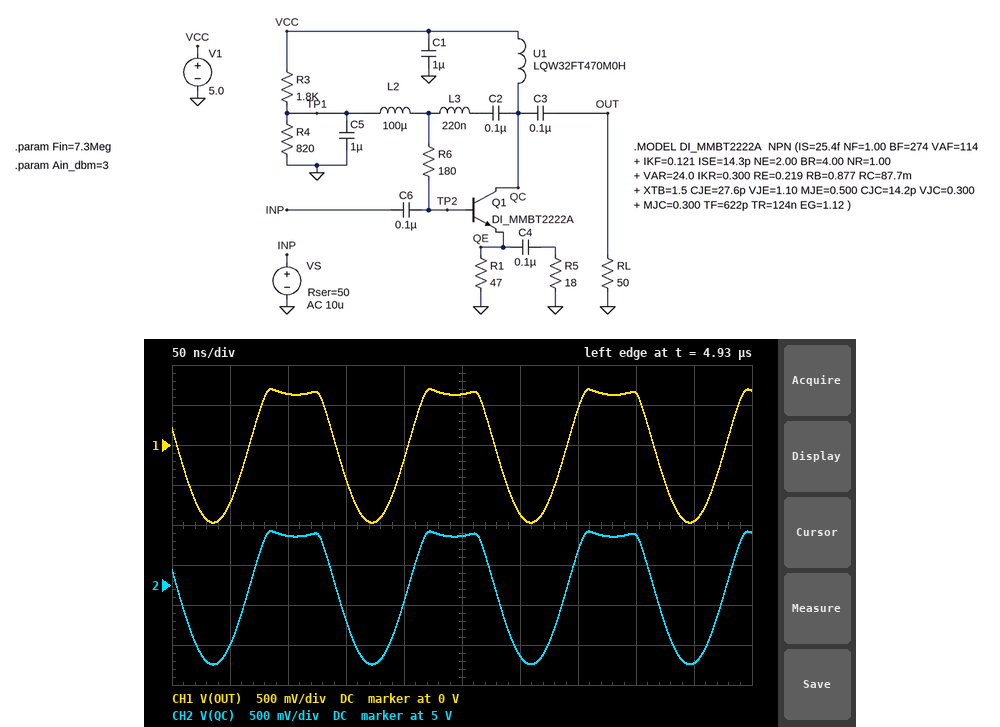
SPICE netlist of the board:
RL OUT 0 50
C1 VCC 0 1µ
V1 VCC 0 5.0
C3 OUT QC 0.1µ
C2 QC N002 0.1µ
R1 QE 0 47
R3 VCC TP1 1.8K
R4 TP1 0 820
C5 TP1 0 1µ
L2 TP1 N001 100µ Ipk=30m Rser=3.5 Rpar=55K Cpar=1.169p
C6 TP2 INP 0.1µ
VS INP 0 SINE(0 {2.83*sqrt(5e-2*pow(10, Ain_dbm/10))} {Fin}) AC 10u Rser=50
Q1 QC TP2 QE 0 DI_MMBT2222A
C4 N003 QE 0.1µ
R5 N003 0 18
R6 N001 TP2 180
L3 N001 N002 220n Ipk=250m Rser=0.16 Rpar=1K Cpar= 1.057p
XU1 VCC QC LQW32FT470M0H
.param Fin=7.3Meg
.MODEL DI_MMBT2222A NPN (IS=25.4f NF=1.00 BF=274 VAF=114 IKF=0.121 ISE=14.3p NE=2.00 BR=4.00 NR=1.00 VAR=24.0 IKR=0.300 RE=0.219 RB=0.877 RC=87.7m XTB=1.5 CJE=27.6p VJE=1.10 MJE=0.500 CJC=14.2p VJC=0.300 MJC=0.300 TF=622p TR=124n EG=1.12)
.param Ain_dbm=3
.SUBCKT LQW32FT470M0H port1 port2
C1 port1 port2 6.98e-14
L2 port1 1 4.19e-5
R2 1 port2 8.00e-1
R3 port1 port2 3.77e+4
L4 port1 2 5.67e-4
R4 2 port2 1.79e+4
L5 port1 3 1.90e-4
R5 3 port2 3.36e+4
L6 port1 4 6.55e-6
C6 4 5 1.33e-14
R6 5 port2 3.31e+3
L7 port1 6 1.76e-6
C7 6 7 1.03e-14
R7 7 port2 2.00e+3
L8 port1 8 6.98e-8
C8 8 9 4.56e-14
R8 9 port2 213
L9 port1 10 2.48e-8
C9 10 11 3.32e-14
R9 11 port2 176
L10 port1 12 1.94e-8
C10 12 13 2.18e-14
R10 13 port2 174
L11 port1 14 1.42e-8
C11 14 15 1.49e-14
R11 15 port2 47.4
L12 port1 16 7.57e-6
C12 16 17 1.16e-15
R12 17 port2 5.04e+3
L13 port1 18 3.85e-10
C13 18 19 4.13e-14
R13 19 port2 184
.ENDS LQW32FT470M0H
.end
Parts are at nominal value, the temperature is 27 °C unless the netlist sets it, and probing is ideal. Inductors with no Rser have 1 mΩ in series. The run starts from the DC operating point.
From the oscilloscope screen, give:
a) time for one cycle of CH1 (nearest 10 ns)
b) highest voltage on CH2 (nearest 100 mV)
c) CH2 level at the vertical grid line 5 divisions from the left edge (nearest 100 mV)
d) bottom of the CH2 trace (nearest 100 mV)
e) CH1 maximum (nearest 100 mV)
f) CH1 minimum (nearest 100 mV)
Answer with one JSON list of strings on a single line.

["140 ns", "5.7 V", "5.6 V", "4.0 V", "700 mV", "-1.0 V"]
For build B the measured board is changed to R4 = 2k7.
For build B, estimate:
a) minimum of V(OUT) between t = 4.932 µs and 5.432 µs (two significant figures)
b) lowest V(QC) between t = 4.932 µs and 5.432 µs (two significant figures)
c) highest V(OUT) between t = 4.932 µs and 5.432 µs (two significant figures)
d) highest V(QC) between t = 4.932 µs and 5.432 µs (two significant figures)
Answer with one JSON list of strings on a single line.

["-1.1 V", "3.8 V", "1.1 V", "6.1 V"]
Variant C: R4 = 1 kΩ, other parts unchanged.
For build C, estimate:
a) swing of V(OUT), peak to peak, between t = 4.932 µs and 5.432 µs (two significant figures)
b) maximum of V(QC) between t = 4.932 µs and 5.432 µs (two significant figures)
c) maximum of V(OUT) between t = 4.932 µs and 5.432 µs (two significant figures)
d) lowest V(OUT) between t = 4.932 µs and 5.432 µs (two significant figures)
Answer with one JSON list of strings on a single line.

["1.8 V", "5.8 V", "800 mV", "-1.0 V"]
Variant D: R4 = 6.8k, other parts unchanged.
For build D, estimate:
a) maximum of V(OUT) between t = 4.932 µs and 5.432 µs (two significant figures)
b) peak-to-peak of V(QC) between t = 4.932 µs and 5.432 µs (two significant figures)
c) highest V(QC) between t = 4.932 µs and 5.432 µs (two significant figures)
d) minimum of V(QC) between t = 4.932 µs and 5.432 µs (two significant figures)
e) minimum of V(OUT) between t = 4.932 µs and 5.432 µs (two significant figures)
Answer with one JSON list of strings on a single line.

["1.1 V", "2.3 V", "6.1 V", "3.8 V", "-1.1 V"]
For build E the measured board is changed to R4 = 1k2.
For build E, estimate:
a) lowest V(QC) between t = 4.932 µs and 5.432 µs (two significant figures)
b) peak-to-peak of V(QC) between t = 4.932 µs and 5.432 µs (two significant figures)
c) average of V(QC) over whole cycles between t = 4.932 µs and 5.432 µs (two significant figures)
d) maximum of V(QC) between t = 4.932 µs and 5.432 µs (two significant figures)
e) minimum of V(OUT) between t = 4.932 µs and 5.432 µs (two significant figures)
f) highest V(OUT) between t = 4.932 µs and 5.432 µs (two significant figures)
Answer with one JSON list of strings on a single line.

["3.9 V", "2.0 V", "5.0 V", "5.9 V", "-1.1 V", "900 mV"]
